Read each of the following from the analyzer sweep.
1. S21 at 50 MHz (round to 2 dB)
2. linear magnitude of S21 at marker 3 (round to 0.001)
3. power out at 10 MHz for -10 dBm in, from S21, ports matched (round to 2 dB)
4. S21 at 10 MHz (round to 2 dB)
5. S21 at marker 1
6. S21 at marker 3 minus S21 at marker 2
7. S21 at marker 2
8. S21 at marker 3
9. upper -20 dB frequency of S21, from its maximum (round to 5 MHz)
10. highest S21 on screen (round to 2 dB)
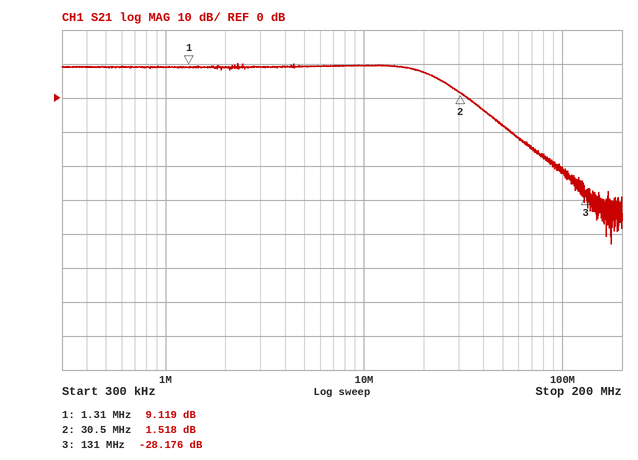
-8 dB
0.039
0 dBm
10 dB
9.119 dB
-29.694 dB
1.518 dB
-28.176 dB
55 MHz
10 dB
